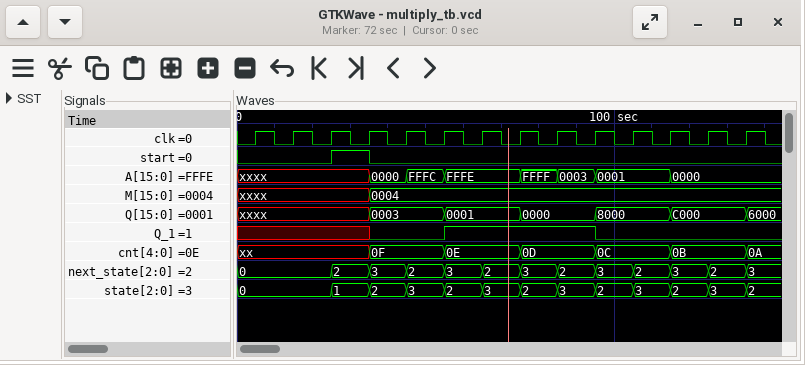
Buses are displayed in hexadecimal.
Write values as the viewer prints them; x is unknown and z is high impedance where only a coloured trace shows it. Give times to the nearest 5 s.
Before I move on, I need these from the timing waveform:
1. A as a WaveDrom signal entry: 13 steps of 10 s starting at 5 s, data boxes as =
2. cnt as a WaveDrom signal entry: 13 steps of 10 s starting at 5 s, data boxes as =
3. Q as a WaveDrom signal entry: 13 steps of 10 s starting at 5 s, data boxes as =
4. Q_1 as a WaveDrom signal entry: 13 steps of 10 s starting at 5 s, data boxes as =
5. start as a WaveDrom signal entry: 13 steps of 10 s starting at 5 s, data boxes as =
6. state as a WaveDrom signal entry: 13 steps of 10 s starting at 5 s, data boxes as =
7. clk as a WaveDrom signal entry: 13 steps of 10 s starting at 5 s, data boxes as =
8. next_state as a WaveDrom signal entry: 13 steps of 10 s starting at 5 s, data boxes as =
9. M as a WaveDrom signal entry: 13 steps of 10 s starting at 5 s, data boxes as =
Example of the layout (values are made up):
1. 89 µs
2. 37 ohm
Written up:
1. {name: 'A', wave: 'x..===.===.=.', data: '0000 FFFC FFFE FFFF 0003 0001 0000'}
2. {name: 'cnt', wave: 'x..=.=.=.=.=.', data: '0F 0E 0D 0C 0B'}
3. {name: 'Q', wave: 'x..=.=.=.=.=.', data: '0003 0001 0000 8000 C000'}
4. {name: 'Q_1', wave: 'x..0.1...0...'}
5. {name: 'start', wave: '0.10.........'}
6. {name: 'state', wave: '=.===========', data: '0 1 2 3 2 3 2 3 2 3 2 3'}
7. {name: 'clk', wave: 'p............'}
8. {name: 'next_state', wave: '=.===========', data: '0 2 3 2 3 2 3 2 3 2 3 2'}
9. {name: 'M', wave: 'x..=.........', data: '0004'}
